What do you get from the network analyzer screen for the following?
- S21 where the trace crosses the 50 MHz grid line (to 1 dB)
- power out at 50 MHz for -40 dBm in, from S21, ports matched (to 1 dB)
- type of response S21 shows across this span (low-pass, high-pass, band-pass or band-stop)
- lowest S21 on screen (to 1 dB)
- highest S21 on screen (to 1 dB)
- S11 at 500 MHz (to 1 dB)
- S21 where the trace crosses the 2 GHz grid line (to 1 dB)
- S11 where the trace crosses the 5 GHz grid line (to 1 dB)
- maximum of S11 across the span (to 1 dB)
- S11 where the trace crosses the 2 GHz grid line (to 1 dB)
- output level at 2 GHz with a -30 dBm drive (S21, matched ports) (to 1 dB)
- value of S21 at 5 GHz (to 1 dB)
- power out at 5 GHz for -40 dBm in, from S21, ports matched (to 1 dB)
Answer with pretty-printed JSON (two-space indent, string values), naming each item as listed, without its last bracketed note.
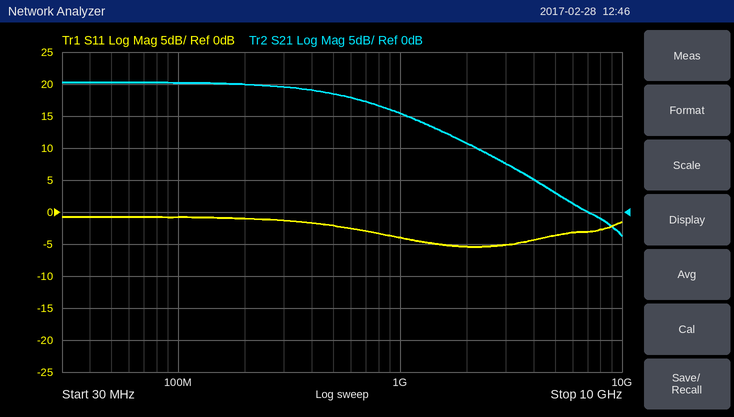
{
  "S21 where the trace crosses the 50 MHz grid line": "20 dB",
  "power out at 50 MHz for -40 dBm in, from S21, ports matched": "-20 dBm",
  "type of response S21 shows across this span": "low-pass",
  "lowest S21 on screen": "-4 dB",
  "highest S21 on screen": "20 dB",
  "S11 at 500 MHz": "-2 dB",
  "S21 where the trace crosses the 2 GHz grid line": "11 dB",
  "S11 where the trace crosses the 5 GHz grid line": "-4 dB",
  "maximum of S11 across the span": "-1 dB",
  "S11 where the trace crosses the 2 GHz grid line": "-5 dB",
  "output level at 2 GHz with a -30 dBm drive (S21, matched ports)": "-19 dBm",
  "value of S21 at 5 GHz": "3 dB",
  "power out at 5 GHz for -40 dBm in, from S21, ports matched": "-37 dBm"
}
